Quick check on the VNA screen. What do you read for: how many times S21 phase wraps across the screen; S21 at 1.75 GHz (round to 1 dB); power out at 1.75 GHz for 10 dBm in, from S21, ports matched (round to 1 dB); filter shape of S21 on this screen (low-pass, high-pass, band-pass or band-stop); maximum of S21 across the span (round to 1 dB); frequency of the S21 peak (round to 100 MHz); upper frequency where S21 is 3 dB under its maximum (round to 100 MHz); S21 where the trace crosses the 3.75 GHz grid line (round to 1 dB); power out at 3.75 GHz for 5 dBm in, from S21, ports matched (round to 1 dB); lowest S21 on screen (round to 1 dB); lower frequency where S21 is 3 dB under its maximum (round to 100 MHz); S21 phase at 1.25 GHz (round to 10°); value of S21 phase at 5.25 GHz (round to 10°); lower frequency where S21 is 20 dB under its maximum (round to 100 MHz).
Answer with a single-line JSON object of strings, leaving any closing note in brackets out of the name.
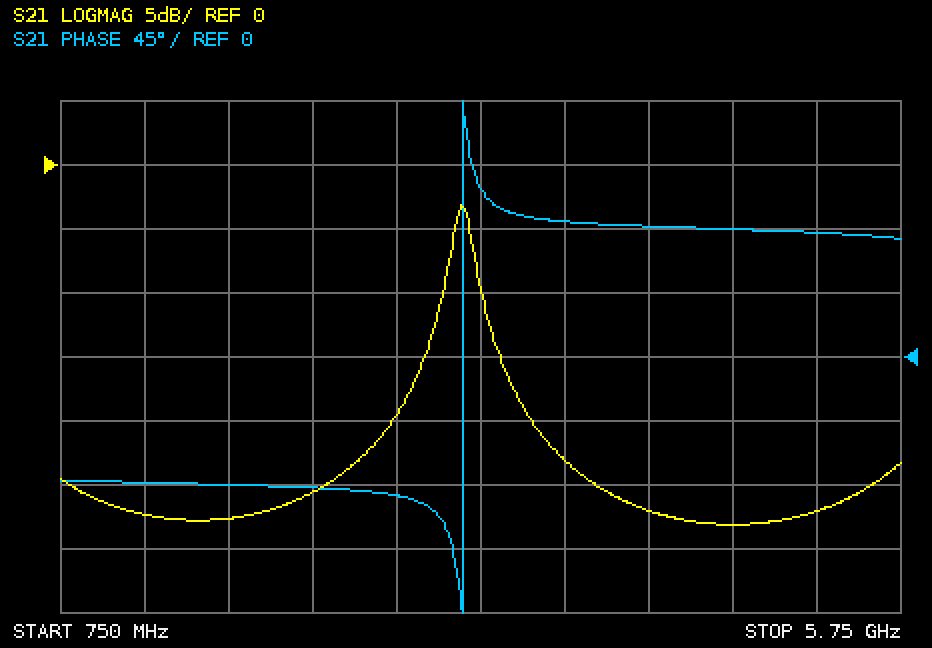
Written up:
{"how many times S21 phase wraps across the screen": "1", "S21 at 1.75 GHz": "-28 dB", "power out at 1.75 GHz for 10 dBm in, from S21, ports matched": "-18 dBm", "filter shape of S21 on this screen": "band-pass", "maximum of S21 across the span": "-3 dB", "frequency of the S21 peak": "3.1 GHz", "upper frequency where S21 is 3 dB under its maximum": "3.2 GHz", "S21 where the trace crosses the 3.75 GHz grid line": "-23 dB", "power out at 3.75 GHz for 5 dBm in, from S21, ports matched": "-18 dBm", "lowest S21 on screen": "-28 dB", "lower frequency where S21 is 3 dB under its maximum": "3.1 GHz", "S21 phase at 1.25 GHz": "-90°", "value of S21 phase at 5.25 GHz": "90°", "lower frequency where S21 is 20 dB under its maximum": "2.5 GHz"}
